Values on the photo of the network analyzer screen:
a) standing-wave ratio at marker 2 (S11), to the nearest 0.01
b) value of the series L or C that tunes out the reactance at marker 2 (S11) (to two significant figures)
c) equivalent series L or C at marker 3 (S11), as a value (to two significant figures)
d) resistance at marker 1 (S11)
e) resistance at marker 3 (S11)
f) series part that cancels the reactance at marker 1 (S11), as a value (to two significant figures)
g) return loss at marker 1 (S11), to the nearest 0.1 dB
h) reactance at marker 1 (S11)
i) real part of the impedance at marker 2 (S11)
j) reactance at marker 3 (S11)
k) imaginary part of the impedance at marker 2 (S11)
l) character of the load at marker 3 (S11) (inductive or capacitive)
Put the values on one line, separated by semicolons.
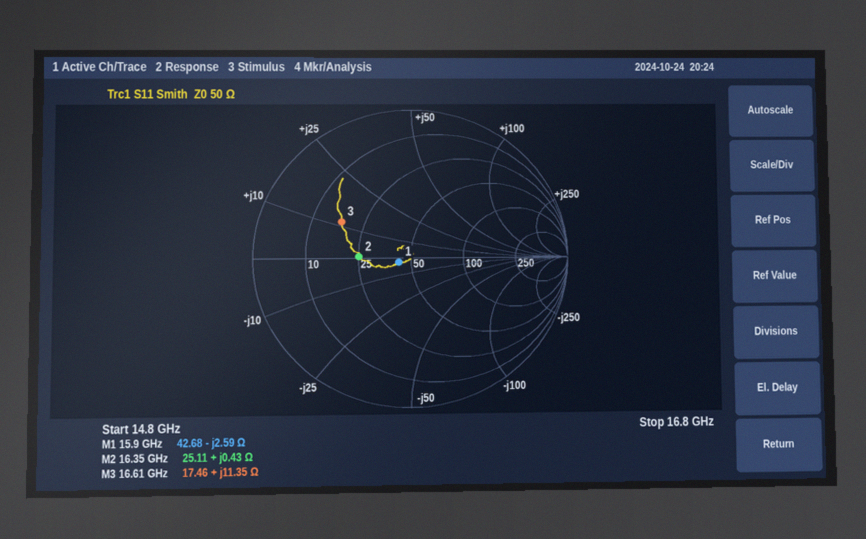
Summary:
1.99; 23 pF; 110 pH; 42.68 Ω; 17.46 Ω; 26 pH; 21.5 dB; -2.59 Ω; 25.11 Ω; +11.35 Ω; +0.43 Ω; inductive
